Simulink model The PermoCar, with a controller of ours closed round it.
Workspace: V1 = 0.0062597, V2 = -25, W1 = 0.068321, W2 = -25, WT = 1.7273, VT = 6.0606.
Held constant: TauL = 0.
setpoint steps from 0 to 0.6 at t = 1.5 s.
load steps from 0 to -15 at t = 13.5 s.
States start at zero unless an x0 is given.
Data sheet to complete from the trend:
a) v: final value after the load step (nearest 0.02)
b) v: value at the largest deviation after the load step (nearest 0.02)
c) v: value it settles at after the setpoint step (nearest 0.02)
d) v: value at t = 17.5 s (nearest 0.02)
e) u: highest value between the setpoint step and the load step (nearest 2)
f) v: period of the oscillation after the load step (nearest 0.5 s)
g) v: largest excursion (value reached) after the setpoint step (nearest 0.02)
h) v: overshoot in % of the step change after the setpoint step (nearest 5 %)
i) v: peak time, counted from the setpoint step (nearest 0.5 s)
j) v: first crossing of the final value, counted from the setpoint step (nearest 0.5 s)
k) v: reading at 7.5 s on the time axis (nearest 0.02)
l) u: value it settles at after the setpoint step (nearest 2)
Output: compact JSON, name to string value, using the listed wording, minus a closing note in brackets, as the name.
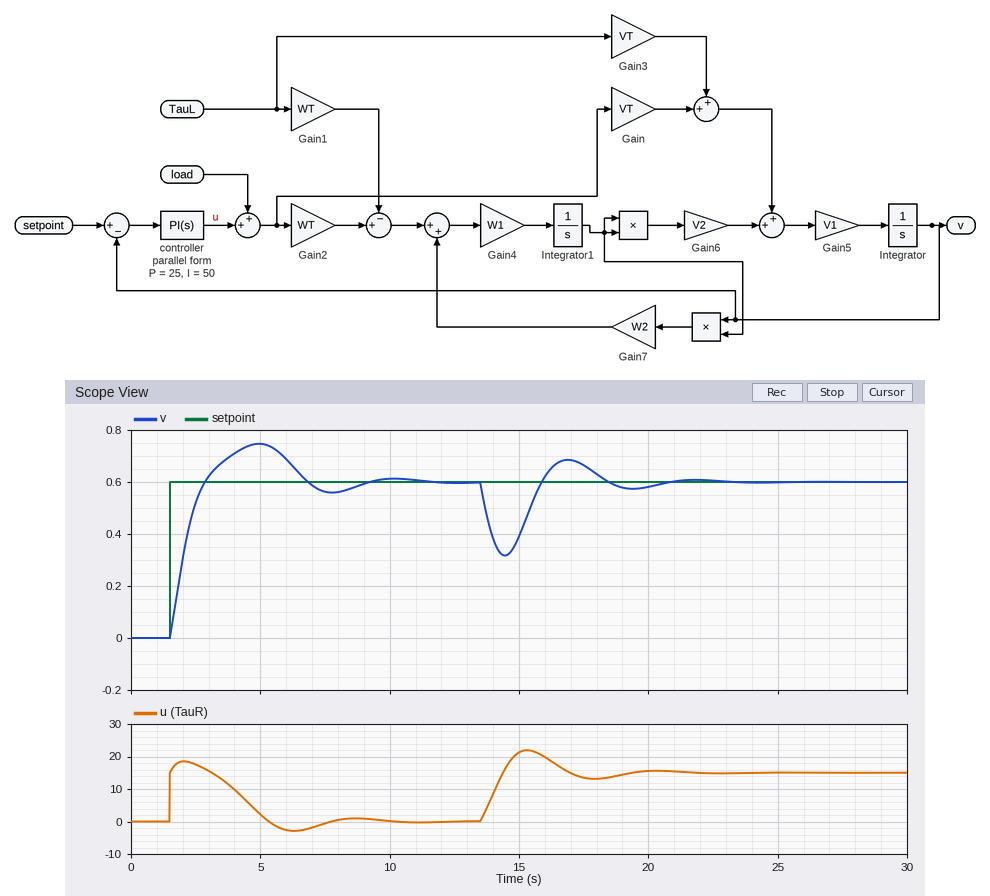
{"v: final value after the load step": "0.60", "v: value at the largest deviation after the load step": "0.32", "v: value it settles at after the setpoint step": "0.60", "v: value at t = 17.5 s": "0.66", "u: highest value between the setpoint step and the load step": "18", "v: period of the oscillation after the load step": "5.0 s", "v: largest excursion (value reached) after the setpoint step": "0.74", "v: overshoot in % of the step change after the setpoint step": "25 %", "v: peak time, counted from the setpoint step": "3.5 s", "v: first crossing of the final value, counted from the setpoint step": "1.5 s", "v: reading at 7.5 s on the time axis": "0.56", "u: value it settles at after the setpoint step": "0"}
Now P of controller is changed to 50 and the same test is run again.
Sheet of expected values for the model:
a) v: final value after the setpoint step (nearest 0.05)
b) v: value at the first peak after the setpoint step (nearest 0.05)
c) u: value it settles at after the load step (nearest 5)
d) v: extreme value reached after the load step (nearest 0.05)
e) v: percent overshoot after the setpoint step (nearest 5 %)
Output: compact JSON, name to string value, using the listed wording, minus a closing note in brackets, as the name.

{"v: final value after the setpoint step": "0.60", "v: value at the first peak after the setpoint step": "0.70", "u: value it settles at after the load step": "15", "v: extreme value reached after the load step": "0.40", "v: percent overshoot after the setpoint step": "15 %"}
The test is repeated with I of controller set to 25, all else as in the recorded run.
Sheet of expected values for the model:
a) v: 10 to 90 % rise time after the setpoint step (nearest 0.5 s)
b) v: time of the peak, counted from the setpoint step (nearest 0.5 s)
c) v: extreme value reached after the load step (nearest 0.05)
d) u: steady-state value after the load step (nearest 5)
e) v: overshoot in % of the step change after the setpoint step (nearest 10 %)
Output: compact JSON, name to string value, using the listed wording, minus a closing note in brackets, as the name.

{"v: 10 to 90 % rise time after the setpoint step": "1.5 s", "v: time of the peak, counted from the setpoint step": "4.5 s", "v: extreme value reached after the load step": "0.25", "u: steady-state value after the load step": "15", "v: overshoot in % of the step change after the setpoint step": "30 %"}
